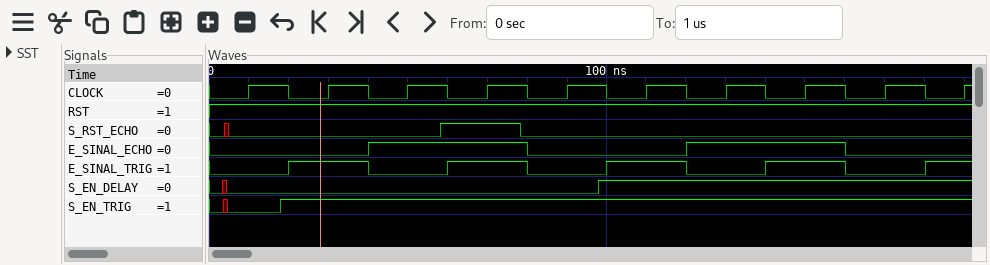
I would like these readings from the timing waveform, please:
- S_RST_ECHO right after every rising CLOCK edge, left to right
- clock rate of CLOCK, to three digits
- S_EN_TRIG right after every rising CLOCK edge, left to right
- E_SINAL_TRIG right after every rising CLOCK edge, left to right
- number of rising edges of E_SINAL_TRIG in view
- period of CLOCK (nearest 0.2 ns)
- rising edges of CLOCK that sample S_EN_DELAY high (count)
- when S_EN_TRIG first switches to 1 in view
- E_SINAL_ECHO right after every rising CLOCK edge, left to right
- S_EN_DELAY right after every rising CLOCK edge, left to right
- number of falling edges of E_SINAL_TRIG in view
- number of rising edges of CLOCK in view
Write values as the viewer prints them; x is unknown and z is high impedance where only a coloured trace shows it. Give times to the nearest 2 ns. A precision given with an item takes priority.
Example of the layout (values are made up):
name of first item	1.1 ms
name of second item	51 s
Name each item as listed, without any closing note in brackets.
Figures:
S_RST_ECHO right after every rising CLOCK edge, left to right	0 0 0 1 0 0 0 0 0 0
clock rate of CLOCK, to three digits	50.0 MHz
S_EN_TRIG right after every rising CLOCK edge, left to right	0 1 1 1 1 1 1 1 1 1
E_SINAL_TRIG right after every rising CLOCK edge, left to right	0 1 0 1 0 1 0 1 0 1
number of rising edges of E_SINAL_TRIG in view	5
period of CLOCK	20 ns
rising edges of CLOCK that sample S_EN_DELAY high	5
when S_EN_TRIG first switches to 1 in view	18 ns
E_SINAL_ECHO right after every rising CLOCK edge, left to right	0 0 1 1 0 0 1 1 0 0
S_EN_DELAY right after every rising CLOCK edge, left to right	0 0 0 0 0 1 1 1 1 1
number of falling edges of E_SINAL_TRIG in view	4
number of rising edges of CLOCK in view	10
